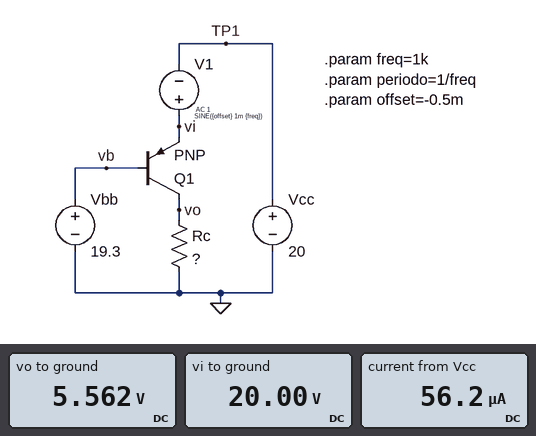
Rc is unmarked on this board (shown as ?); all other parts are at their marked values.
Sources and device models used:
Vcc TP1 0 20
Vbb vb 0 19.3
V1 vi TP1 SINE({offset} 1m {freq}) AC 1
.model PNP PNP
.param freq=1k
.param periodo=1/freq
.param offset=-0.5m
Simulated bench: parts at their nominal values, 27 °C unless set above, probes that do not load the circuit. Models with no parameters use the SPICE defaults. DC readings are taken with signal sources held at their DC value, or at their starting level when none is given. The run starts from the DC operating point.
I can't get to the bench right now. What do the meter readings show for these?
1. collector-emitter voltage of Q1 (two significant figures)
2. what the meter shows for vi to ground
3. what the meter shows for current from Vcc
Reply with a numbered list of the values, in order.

1. -14 V
2. 20.00 V
3. 56.2 µA
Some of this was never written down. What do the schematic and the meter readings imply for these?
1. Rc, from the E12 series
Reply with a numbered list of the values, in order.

1. 100 kΩ
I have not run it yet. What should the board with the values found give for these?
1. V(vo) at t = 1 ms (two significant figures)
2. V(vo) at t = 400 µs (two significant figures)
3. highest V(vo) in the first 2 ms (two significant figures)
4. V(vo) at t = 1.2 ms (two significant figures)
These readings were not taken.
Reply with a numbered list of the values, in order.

1. 5.6 V
2. 5.7 V
3. 5.8 V
4. 5.8 V
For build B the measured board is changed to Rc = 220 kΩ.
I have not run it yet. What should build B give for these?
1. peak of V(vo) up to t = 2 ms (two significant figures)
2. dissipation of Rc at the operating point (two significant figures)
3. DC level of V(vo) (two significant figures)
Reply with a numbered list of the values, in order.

1. 13 V
2. 680 µW
3. 12 V
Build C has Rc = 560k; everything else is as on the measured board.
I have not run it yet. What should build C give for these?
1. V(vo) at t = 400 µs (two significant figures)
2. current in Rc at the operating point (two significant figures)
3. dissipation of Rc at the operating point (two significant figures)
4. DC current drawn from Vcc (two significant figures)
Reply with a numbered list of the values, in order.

1. 20 V
2. 36 µA
3. 710 µW
4. 46 µA
